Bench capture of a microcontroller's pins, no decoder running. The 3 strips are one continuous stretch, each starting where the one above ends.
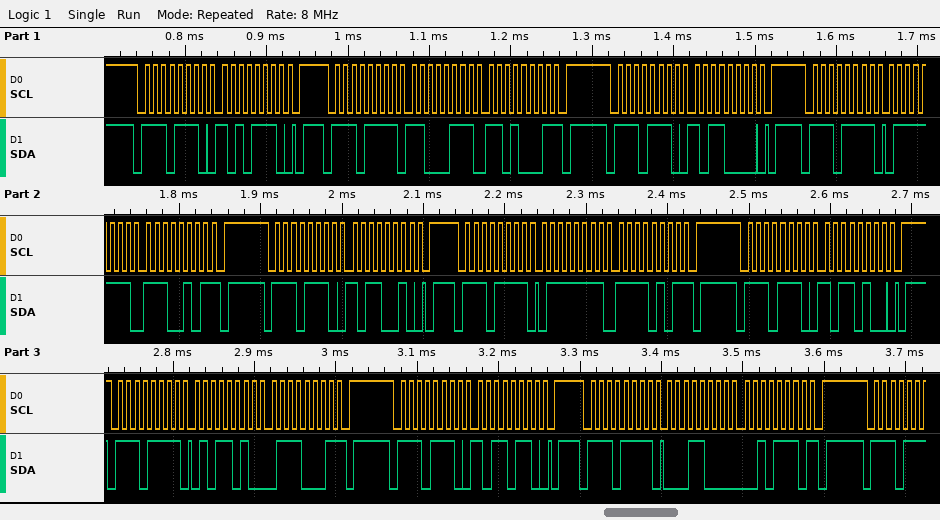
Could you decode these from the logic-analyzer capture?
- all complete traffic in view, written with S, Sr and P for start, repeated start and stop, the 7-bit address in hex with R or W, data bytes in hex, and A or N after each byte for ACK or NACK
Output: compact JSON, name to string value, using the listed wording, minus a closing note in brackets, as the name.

{"all complete traffic in view, written with S, Sr and P for start, repeated start and stop, the 7-bit address in hex with R or W, data bytes in hex, and A or N after each byte for ACK or NACK": "S 77W A AE A P S 77R A C7 A D1 N P S 77W A B0 A P S 77R A 7F A E5 N P S 77W A B2 A P S 77R A 7F A F5 N P S 77W A B4 A P S 77R A 5A A 71 N P S 77W A B6 A P S 77R A 18 A 2E N P"}
